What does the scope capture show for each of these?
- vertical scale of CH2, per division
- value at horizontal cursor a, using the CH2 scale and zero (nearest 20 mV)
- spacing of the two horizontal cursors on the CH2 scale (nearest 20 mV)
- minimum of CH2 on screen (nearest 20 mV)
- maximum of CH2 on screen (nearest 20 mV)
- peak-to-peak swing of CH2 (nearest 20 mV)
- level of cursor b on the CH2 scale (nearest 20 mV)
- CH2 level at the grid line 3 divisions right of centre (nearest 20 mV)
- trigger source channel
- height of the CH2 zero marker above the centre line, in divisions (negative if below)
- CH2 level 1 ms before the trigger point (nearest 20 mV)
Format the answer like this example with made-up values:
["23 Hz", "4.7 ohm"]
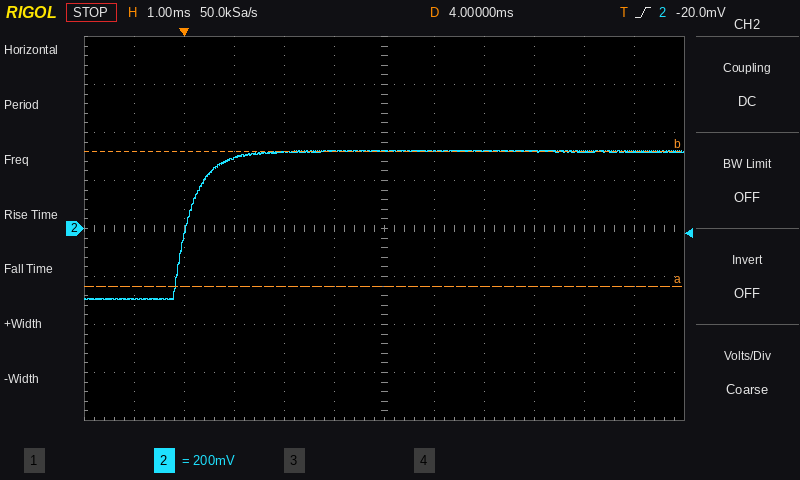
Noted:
["200 mV", "-240 mV", "560 mV", "-300 mV", "320 mV", "620 mV", "320 mV", "320 mV", "CH2", "0.0 div", "-300 mV"]
